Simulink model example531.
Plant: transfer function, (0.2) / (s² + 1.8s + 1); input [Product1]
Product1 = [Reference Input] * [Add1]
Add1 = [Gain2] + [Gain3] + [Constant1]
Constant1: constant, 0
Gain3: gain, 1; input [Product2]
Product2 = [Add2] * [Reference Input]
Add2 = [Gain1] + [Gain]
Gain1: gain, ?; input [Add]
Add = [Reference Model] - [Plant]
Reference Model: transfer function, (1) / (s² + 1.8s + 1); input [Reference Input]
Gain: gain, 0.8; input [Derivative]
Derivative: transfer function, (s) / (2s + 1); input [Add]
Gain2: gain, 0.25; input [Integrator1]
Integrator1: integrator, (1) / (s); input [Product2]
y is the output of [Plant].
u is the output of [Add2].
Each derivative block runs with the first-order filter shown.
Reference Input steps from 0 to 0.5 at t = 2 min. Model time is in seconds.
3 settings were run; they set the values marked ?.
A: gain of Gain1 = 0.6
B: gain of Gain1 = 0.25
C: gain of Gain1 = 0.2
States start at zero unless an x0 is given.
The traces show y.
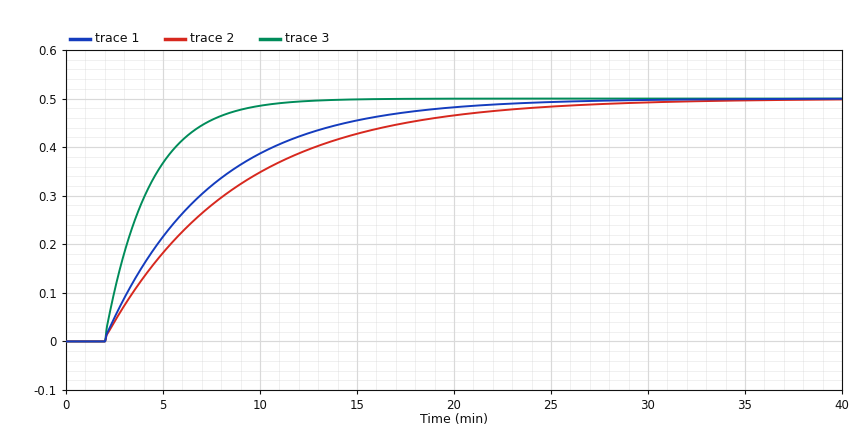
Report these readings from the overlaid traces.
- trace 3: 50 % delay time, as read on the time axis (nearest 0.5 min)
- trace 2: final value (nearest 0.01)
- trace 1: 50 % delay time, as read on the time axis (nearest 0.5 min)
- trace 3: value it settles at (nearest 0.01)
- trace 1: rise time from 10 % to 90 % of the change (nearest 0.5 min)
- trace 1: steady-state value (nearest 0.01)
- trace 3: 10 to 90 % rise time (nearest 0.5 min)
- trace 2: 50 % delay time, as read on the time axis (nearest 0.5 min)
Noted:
3.5 min
0.50
5.5 min
0.50
12.0 min
0.50
5.0 min
6.5 min
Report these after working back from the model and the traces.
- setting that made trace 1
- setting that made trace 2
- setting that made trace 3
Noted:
B
C
A
